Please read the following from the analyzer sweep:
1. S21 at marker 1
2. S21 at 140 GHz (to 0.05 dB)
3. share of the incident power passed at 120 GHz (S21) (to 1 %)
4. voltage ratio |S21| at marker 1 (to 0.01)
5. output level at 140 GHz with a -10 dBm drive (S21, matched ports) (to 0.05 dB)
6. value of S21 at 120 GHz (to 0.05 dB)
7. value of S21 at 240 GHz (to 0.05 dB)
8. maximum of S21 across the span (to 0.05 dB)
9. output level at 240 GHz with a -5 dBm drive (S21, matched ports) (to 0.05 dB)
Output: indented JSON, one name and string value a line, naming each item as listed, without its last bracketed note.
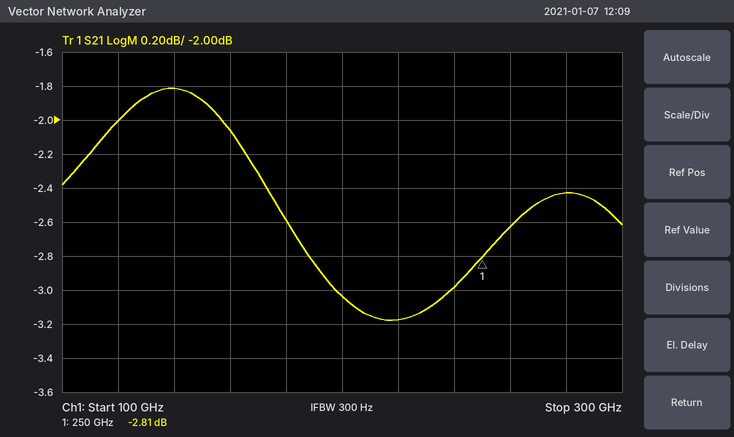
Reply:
{
  "S21 at marker 1": "-2.81 dB",
  "S21 at 140 GHz": "-1.80 dB",
  "share of the incident power passed at 120 GHz (S21)": "63 %",
  "voltage ratio |S21| at marker 1": "0.72",
  "output level at 140 GHz with a -10 dBm drive (S21, matched ports)": "-11.80 dBm",
  "value of S21 at 120 GHz": "-2.00 dB",
  "value of S21 at 240 GHz": "-3.00 dB",
  "maximum of S21 across the span": "-1.80 dB",
  "output level at 240 GHz with a -5 dBm drive (S21, matched ports)": "-8.00 dBm"
}
